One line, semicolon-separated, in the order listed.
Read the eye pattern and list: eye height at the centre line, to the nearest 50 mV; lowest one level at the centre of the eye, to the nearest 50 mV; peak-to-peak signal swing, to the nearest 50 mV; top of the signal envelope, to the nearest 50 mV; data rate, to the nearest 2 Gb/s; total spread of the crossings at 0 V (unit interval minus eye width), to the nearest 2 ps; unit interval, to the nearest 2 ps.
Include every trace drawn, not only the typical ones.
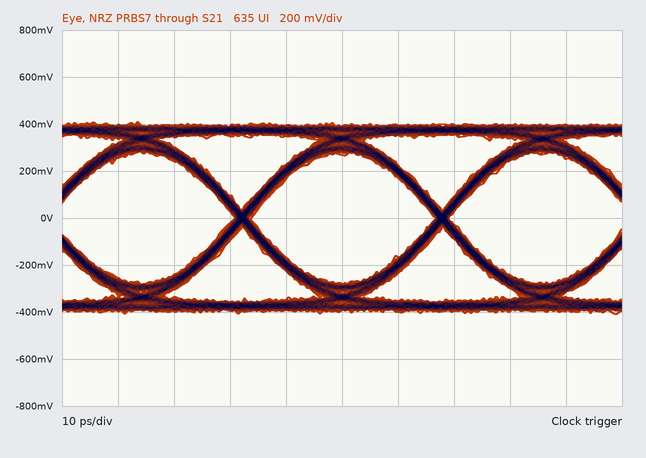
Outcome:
550 mV; 250 mV; 800 mV; 400 mV; 28 Gb/s; 2 ps; 36 ps
